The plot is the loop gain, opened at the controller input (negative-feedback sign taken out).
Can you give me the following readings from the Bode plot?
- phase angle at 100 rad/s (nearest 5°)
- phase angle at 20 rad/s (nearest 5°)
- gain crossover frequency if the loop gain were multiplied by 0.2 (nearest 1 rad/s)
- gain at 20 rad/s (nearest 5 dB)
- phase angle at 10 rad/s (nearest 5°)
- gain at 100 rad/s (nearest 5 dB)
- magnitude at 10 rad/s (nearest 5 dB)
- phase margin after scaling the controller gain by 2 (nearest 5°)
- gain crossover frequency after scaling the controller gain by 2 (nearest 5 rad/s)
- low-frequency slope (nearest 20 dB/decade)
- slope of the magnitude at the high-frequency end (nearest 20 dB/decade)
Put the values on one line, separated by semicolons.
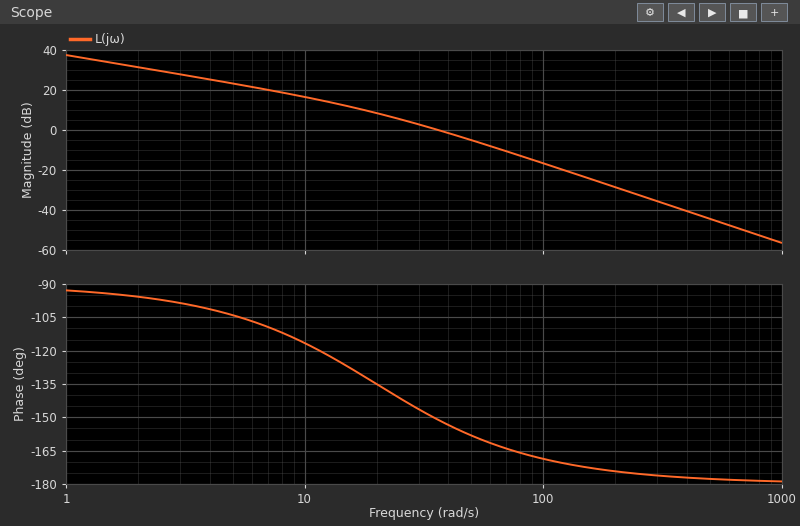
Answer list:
-170°; -135°; 13 rad/s; 10 dB; -115°; -15 dB; 15 dB; 20°; 55 rad/s; -20 dB/decade; -40 dB/decade
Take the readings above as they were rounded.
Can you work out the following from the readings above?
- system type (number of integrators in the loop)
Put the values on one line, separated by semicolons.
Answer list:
1
